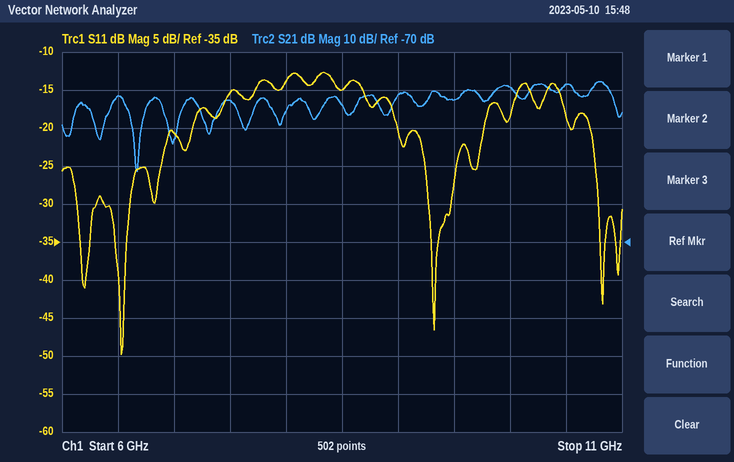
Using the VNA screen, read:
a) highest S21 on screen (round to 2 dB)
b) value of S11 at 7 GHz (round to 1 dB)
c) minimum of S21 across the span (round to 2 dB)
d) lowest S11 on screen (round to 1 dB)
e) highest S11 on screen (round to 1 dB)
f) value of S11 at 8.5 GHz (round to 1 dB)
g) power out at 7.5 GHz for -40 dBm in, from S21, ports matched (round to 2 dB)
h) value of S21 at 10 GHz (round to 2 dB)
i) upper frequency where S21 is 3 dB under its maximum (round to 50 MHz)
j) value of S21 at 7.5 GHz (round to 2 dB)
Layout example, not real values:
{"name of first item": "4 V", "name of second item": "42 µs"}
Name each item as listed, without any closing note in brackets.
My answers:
{"highest S21 on screen": "-28 dB", "value of S11 at 7 GHz": "-21 dB", "minimum of S21 across the span": "-52 dB", "lowest S11 on screen": "-50 dB", "highest S11 on screen": "-13 dB", "value of S11 at 8.5 GHz": "-15 dB", "power out at 7.5 GHz for -40 dBm in, from S21, ports matched": "-72 dBm", "value of S21 at 10 GHz": "-30 dB", "upper frequency where S21 is 3 dB under its maximum": "10.90 GHz", "value of S21 at 7.5 GHz": "-32 dB"}
